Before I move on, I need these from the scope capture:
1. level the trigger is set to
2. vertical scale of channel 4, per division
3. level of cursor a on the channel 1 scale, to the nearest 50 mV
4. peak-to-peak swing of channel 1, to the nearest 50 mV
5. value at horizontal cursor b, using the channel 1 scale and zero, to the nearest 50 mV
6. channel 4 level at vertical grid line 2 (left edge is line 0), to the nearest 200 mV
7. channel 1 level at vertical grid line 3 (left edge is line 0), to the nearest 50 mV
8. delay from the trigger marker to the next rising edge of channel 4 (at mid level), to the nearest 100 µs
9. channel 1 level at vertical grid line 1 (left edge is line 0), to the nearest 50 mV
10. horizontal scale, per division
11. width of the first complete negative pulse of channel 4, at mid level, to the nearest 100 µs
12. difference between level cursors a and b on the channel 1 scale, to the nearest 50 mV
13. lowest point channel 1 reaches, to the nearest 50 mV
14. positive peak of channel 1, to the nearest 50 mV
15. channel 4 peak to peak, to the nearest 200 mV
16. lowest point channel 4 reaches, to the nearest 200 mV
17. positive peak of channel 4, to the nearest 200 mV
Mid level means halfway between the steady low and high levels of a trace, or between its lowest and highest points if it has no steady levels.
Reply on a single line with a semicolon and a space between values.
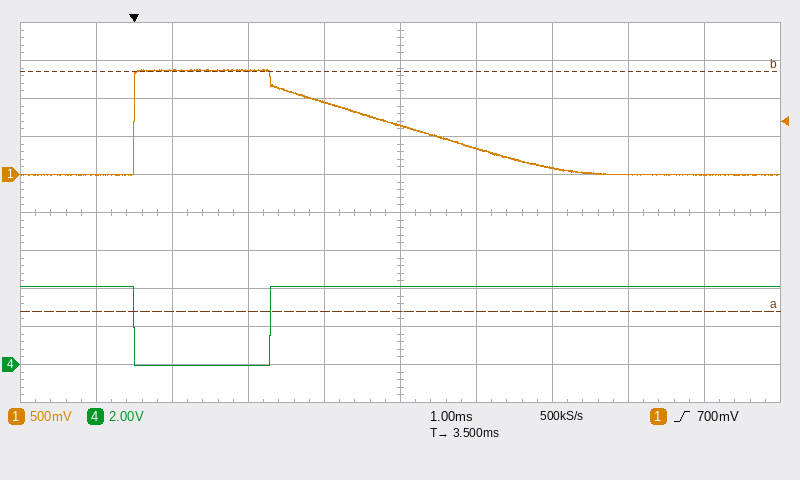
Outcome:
700 mV; 2 V; -1.80 V; 1.40 V; 1.35 V; 0.0 V; 1.35 V; 1.8 ms; 0 mV; 1 ms; 1.8 ms; 3.15 V; 0 mV; 1.40 V; 4.2 V; 0.0 V; 4.2 V
